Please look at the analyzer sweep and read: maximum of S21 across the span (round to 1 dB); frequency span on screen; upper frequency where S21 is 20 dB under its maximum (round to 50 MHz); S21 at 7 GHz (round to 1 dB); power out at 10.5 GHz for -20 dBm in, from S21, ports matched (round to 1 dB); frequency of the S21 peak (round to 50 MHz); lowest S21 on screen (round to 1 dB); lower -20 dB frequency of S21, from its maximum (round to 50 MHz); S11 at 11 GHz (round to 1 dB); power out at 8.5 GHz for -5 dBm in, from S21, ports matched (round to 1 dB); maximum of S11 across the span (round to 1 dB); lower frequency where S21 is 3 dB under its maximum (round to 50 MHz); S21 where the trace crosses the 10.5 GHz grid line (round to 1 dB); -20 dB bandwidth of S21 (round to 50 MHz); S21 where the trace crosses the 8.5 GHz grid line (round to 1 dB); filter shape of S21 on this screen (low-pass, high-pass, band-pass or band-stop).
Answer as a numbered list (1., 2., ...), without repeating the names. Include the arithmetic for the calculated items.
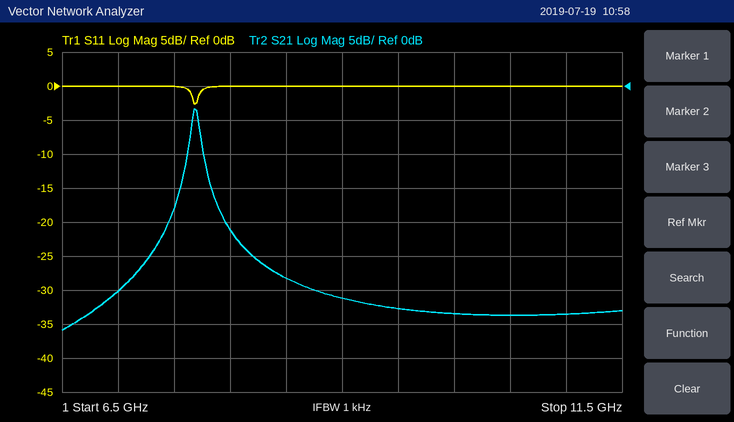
1. -3 dB
2. 5 GHz
3. 8.10 GHz
4. -30 dB
5. -20 dBm + (-34 dB) = -54 dBm
6. 7.70 GHz
7. -36 dB
8. 7.35 GHz
9. 0 dB
10. -5 dBm + (-28 dB) = -33 dBm
11. 0 dB
12. 7.65 GHz
13. -34 dB
14. 8.10 GHz − 7.35 GHz = 750 MHz
15. -28 dB
16. band-pass
